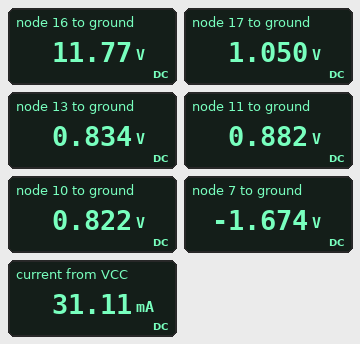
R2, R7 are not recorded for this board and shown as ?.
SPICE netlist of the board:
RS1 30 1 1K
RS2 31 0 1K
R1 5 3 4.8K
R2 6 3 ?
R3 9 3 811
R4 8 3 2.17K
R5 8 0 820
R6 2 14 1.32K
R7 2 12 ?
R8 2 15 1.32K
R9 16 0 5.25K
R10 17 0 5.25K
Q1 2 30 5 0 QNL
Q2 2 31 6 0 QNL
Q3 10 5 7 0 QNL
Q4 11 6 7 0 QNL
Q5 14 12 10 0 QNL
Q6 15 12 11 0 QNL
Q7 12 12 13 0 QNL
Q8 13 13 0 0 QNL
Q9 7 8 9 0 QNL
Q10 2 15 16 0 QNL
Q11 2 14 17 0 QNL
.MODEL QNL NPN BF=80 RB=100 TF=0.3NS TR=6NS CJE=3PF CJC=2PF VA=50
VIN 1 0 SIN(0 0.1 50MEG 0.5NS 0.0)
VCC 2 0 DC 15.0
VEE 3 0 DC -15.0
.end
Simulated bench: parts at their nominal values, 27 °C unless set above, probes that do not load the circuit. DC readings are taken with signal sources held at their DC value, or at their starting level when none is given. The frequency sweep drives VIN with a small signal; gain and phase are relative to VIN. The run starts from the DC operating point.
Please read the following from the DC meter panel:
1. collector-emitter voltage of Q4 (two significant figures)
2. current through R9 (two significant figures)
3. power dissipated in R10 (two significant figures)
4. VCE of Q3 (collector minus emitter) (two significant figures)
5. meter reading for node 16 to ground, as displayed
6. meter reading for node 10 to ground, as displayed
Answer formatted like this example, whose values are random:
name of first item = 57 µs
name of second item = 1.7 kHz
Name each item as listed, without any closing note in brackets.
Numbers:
collector-emitter voltage of Q4 = 2.6 V
current through R9 = 2.2 mA
power dissipated in R10 = 210 µW
VCE of Q3 (collector minus emitter) = 2.5 V
meter reading for node 16 to ground, as displayed = 11.77 V
meter reading for node 10 to ground, as displayed = 0.822 V
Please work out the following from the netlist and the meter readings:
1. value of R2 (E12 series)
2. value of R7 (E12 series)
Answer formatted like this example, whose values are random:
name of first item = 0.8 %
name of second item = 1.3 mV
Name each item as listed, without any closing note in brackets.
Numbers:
value of R2 = 2.2 kΩ
value of R7 = 1.8 kΩ
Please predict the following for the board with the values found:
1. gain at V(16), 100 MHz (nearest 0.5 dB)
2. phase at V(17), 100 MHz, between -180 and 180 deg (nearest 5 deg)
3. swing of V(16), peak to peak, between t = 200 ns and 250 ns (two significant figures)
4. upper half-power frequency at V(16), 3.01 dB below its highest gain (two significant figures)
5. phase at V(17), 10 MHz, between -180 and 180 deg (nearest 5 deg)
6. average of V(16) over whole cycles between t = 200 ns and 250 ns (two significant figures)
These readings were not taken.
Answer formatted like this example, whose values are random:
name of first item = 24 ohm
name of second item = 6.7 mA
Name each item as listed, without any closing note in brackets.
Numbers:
gain at V(16), 100 MHz = 11.0 dB
phase at V(17), 100 MHz, between -180 and 180 deg = -40 deg
swing of V(16), peak to peak, between t = 200 ns and 250 ns = 4.5 V
upper half-power frequency at V(16), 3.01 dB below its highest gain = 33 MHz
phase at V(17), 10 MHz, between -180 and 180 deg = 145 deg
average of V(16) over whole cycles between t = 200 ns and 250 ns = 11 V
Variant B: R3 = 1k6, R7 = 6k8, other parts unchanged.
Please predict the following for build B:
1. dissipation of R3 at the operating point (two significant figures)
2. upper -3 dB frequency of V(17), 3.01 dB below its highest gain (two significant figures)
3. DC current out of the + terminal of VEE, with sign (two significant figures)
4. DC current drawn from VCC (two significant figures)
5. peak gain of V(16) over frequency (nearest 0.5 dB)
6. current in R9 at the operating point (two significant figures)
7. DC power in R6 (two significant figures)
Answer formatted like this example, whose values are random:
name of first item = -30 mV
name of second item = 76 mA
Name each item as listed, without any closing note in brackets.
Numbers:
dissipation of R3 at the operating point = 63 mW
upper -3 dB frequency of V(17), 3.01 dB below its highest gain = 47 MHz
DC current out of the + terminal of VEE, with sign = -21 mA
DC current drawn from VCC = 21 mA
peak gain of V(16) over frequency = 30.0 dB
current in R9 at the operating point = 2.5 mA
DC power in R6 = 37 mW
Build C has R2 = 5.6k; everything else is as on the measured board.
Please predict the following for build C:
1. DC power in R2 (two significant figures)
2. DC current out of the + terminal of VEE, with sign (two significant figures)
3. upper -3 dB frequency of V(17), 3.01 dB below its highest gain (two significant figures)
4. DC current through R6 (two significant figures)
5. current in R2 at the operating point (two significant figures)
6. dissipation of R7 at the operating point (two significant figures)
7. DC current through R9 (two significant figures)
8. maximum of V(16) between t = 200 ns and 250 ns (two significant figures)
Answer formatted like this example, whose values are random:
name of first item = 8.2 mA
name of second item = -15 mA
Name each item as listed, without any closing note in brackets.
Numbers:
DC power in R2 = 36 mW
DC current out of the + terminal of VEE, with sign = -23 mA
upper -3 dB frequency of V(17), 3.01 dB below its highest gain = 24 MHz
DC current through R6 = 5.2 mA
current in R2 at the operating point = 2.5 mA
dissipation of R7 at the operating point = 99 mW
DC current through R9 = 1.0 mA
maximum of V(16) between t = 200 ns and 250 ns = 7.9 V
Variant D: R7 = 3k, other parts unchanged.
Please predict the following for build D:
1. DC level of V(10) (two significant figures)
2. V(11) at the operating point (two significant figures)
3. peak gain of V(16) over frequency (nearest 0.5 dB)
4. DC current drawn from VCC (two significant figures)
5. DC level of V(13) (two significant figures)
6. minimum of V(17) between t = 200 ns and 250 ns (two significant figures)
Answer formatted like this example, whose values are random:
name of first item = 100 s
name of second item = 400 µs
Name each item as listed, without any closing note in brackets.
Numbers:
DC level of V(10) = 790 mV
V(11) at the operating point = 850 mV
peak gain of V(16) over frequency = 36.5 dB
DC current drawn from VCC = 28 mA
DC level of V(13) = 820 mV
minimum of V(17) between t = 200 ns and 250 ns = 170 mV
